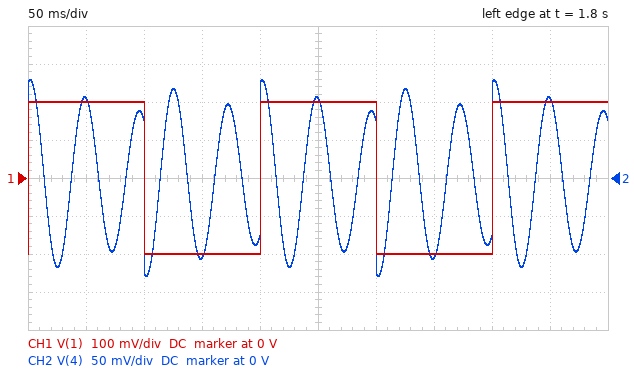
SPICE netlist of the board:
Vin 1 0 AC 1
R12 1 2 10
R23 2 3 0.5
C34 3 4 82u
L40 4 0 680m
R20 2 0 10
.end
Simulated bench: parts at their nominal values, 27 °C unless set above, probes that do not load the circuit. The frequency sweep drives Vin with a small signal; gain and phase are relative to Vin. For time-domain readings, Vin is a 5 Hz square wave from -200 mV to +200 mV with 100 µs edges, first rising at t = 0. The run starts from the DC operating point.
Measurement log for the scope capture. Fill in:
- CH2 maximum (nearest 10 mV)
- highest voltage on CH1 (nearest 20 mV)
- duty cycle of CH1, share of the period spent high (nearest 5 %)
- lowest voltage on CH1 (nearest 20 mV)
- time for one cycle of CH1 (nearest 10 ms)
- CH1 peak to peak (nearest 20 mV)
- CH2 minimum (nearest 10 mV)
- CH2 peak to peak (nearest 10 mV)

130 mV
200 mV
50 %
-200 mV
200 ms
400 mV
-130 mV
260 mV
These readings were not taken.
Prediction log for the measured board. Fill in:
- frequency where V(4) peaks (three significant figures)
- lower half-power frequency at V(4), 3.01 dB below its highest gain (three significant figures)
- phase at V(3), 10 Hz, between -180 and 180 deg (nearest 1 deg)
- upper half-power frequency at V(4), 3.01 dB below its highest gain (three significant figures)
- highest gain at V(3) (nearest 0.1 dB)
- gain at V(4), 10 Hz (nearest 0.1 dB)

21.3 Hz
20.7 Hz
-2 deg
22.0 Hz
-6.0 dB
-17.0 dB
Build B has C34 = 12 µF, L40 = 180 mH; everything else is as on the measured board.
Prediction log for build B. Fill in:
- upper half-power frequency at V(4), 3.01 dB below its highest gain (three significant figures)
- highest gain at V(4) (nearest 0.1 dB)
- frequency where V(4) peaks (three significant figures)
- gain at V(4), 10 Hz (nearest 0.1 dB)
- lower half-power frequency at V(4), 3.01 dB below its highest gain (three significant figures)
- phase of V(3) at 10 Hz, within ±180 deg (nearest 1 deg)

111 Hz
20.9 dB
108 Hz
-47.3 dB
106 Hz
0 deg
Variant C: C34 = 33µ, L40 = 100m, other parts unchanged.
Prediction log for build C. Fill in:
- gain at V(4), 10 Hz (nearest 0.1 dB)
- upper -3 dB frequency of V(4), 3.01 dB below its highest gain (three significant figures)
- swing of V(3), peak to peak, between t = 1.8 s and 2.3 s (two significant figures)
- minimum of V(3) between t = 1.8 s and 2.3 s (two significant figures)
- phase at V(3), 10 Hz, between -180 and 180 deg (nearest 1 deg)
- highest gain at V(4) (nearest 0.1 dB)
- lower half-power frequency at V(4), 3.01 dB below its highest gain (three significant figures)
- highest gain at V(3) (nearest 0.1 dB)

-43.6 dB
92.6 Hz
230 mV
-120 mV
-1 deg
14.0 dB
83.7 Hz
-6.0 dB
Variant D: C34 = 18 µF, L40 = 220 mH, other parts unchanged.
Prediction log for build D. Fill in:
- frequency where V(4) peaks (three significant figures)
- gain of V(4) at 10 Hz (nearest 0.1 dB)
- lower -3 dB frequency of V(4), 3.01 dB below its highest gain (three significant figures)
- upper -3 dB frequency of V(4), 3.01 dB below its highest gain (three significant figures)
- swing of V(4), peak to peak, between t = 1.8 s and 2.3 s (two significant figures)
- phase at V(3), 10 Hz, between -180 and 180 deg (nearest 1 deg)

80.0 Hz
-42.0 dB
78.1 Hz
82.1 Hz
310 mV
0 deg
